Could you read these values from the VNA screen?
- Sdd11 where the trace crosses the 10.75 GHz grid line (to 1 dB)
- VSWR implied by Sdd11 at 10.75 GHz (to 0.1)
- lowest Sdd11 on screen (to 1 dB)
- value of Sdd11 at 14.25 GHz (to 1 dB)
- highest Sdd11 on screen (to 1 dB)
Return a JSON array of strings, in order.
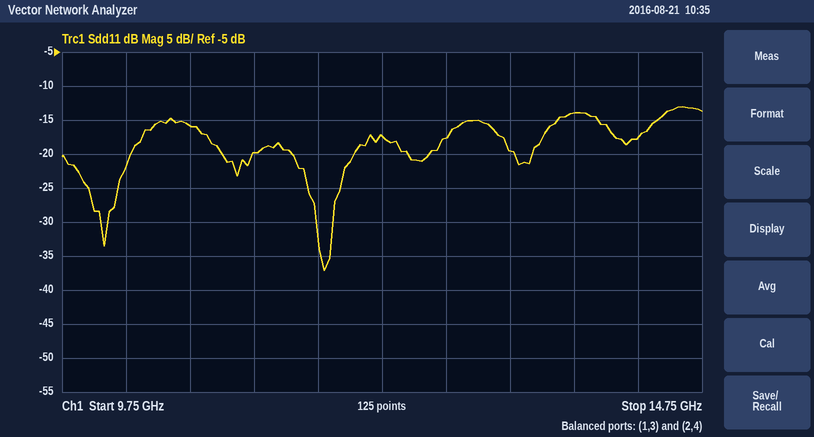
["-16 dB", "1.4", "-37 dB", "-18 dB", "-13 dB"]
